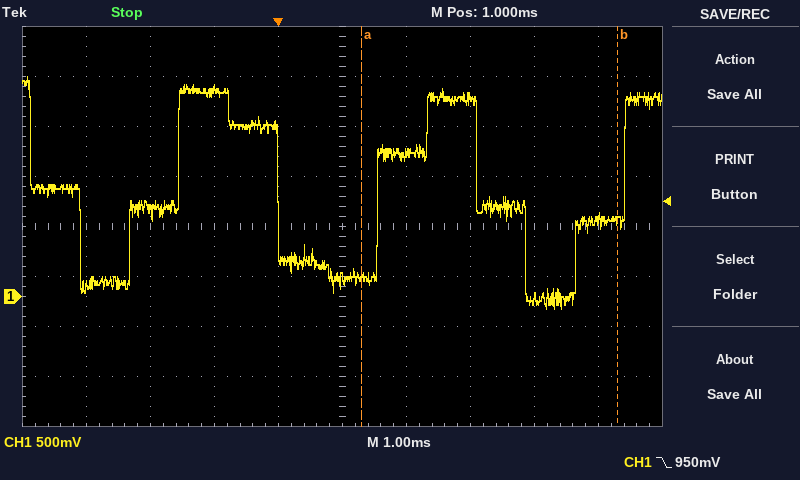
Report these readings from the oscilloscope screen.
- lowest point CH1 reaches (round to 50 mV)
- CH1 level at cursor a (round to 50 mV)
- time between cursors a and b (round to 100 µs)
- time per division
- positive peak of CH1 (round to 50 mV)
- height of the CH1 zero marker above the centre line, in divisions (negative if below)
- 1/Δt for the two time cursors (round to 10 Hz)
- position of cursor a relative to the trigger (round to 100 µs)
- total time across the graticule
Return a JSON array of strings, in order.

["-100 mV", "200 mV", "4.0 ms", "1 ms", "2.20 V", "-1.4 div", "250 Hz", "+1.3 ms", "10 ms"]
